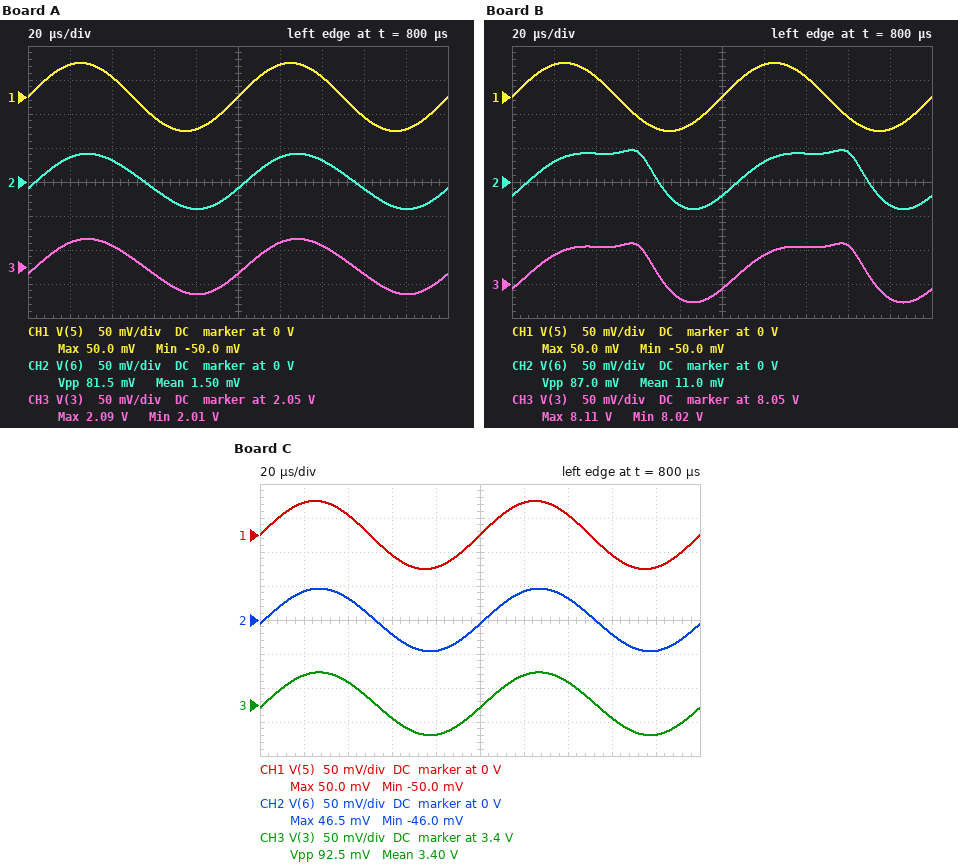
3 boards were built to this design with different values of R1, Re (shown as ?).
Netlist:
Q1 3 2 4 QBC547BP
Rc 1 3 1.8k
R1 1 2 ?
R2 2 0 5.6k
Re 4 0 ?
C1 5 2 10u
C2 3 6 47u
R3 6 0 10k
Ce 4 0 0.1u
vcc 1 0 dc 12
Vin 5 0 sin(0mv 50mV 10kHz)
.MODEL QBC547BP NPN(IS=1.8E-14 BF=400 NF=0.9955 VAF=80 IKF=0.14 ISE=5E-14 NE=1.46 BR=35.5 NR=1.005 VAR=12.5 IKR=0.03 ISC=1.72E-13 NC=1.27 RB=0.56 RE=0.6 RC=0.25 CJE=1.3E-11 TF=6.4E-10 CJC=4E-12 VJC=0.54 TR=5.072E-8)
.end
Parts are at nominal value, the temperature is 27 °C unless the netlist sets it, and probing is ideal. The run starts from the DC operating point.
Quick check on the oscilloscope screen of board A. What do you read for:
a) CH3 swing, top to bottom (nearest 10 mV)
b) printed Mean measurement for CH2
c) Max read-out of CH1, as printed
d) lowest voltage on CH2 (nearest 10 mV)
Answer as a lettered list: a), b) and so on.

a) 80 mV
b) 1.50 mV
c) 50.0 mV
d) -40 mV
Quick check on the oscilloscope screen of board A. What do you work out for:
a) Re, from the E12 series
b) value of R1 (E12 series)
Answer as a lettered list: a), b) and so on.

a) 330 Ω
b) 8.2 kΩ
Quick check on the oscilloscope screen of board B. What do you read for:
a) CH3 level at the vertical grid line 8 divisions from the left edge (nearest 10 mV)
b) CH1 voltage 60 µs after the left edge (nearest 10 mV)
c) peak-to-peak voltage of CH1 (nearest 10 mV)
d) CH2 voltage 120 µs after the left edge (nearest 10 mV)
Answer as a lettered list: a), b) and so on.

a) 8.11 V
b) -30 mV
c) 100 mV
d) 30 mV
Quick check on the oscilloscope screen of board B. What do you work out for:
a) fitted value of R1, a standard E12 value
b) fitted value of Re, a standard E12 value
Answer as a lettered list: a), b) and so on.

a) 1.8 kΩ
b) 3.3 kΩ
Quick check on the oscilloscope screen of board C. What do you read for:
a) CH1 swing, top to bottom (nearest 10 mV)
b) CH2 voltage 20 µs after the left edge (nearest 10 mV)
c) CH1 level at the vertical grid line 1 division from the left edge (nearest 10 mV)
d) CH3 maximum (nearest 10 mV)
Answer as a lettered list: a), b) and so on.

a) 100 mV
b) 40 mV
c) 50 mV
d) 3.45 V
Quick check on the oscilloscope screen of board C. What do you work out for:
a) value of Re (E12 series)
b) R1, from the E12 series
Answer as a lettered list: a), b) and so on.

a) 560 Ω
b) 3.9 kΩ
